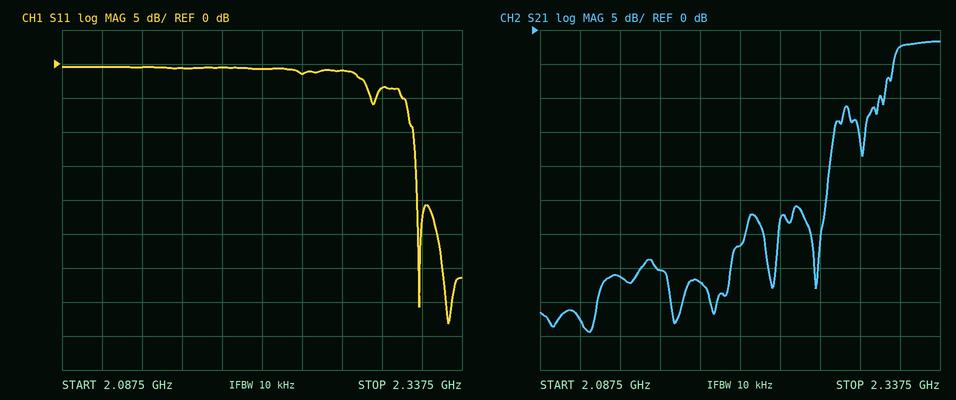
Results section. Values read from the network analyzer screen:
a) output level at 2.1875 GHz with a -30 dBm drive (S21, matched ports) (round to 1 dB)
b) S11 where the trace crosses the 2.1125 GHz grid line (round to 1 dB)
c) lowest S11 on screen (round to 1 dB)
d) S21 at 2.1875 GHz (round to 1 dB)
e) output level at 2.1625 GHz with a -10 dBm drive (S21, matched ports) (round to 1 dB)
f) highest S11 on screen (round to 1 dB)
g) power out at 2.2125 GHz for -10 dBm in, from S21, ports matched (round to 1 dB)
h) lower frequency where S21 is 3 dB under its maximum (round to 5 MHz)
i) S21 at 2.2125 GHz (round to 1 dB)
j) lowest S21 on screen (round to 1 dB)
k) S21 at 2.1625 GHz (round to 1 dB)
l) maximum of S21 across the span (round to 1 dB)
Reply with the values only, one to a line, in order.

-67 dBm
0 dB
-38 dB
-37 dB
-45 dBm
0 dB
-42 dBm
2.310 GHz
-32 dB
-44 dB
-35 dB
-2 dB
